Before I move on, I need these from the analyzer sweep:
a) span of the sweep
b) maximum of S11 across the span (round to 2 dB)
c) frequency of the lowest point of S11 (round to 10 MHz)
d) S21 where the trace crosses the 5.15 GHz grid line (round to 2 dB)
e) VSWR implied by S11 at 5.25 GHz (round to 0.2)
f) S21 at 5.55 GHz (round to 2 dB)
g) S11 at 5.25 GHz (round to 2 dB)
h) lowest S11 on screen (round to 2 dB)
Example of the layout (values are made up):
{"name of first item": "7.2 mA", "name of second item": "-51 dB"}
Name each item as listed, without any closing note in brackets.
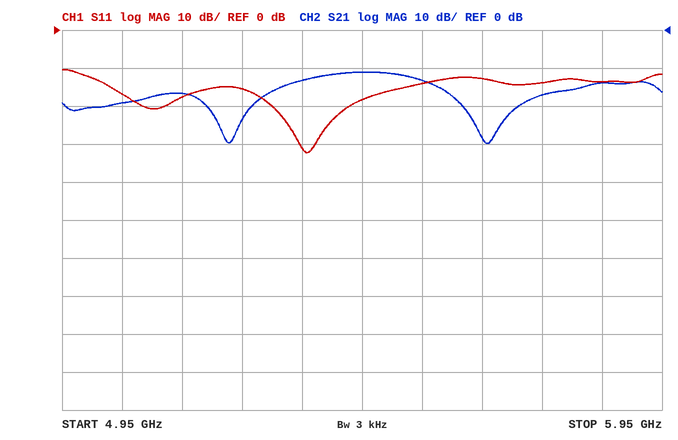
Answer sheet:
{"span of the sweep": "1 GHz", "maximum of S11 across the span": "-10 dB", "frequency of the lowest point of S11": "5.36 GHz", "S21 where the trace crosses the 5.15 GHz grid line": "-16 dB", "VSWR implied by S11 at 5.25 GHz": "1.4", "S21 at 5.55 GHz": "-14 dB", "S11 at 5.25 GHz": "-16 dB", "lowest S11 on screen": "-32 dB"}
